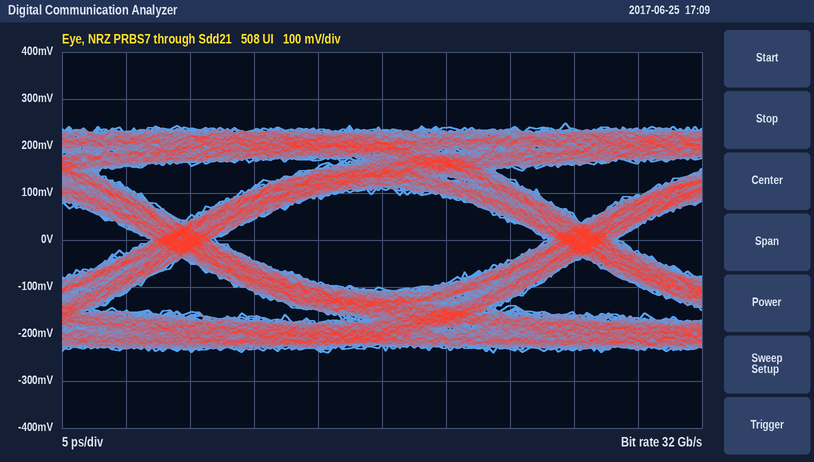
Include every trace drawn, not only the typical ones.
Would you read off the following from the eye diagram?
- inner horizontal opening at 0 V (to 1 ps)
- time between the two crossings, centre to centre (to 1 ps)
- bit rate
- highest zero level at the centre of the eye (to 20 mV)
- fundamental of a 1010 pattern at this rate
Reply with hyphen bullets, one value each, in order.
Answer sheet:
- 26 ps
- 31 ps
- 32 Gb/s
- -100 mV
- 16 GHz
